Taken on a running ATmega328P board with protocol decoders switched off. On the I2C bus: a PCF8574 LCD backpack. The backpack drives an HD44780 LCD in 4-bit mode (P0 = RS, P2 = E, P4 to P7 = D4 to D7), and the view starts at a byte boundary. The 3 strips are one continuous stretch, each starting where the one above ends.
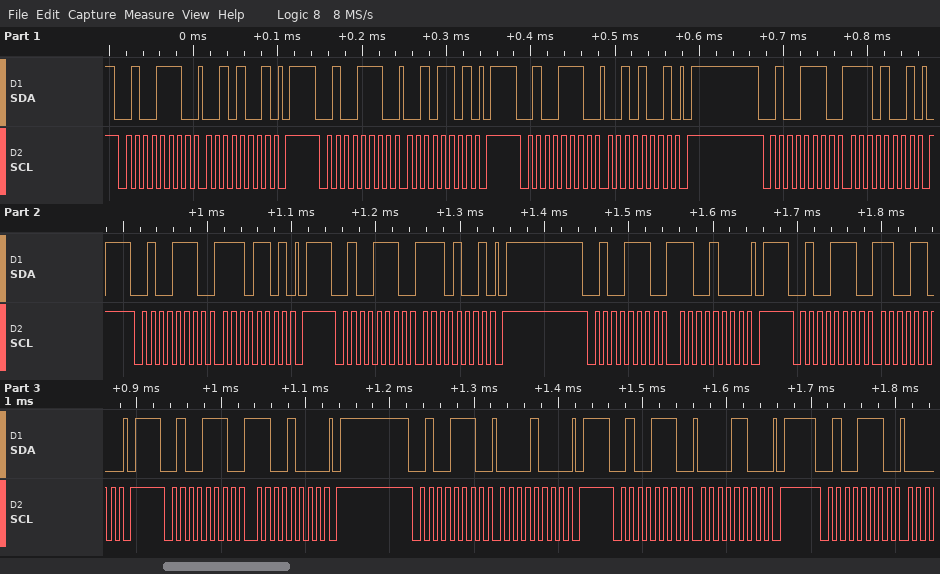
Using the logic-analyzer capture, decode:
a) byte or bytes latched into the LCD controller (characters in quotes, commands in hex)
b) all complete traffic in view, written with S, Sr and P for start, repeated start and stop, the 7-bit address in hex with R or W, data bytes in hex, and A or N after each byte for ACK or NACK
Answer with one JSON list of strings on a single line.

["'.'", "S 27W A 29 A P S 27W A 2D A P S 27W A 29 A P S 27W A E9 A P S 27W A ED A P S 27W A E9 A P S 27W A C8 A P S 27W A CC A P S 27W A C8 A P S 27W A 08 A P S 27W A 0C A P S 27W A"]
